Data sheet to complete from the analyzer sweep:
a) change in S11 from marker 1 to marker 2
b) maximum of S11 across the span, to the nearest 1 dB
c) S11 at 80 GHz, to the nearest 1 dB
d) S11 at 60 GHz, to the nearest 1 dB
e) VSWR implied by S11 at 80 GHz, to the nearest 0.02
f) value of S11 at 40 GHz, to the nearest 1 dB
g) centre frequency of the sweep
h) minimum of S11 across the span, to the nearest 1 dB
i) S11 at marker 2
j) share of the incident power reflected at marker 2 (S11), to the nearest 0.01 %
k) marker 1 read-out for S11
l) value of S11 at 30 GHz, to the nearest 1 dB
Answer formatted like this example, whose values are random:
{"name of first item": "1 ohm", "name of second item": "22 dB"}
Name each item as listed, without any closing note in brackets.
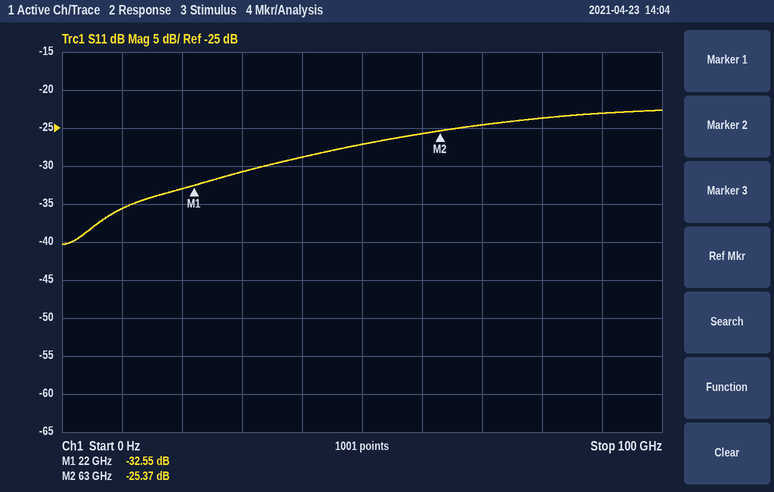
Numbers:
{"change in S11 from marker 1 to marker 2": "7.18 dB", "maximum of S11 across the span, to the nearest 1 dB": "-23 dB", "S11 at 80 GHz, to the nearest 1 dB": "-24 dB", "S11 at 60 GHz, to the nearest 1 dB": "-26 dB", "VSWR implied by S11 at 80 GHz, to the nearest 0.02": "1.14", "value of S11 at 40 GHz, to the nearest 1 dB": "-29 dB", "centre frequency of the sweep": "50 GHz", "minimum of S11 across the span, to the nearest 1 dB": "-40 dB", "S11 at marker 2": "-25.37 dB", "share of the incident power reflected at marker 2 (S11), to the nearest 0.01 %": "0.29 %", "marker 1 read-out for S11": "-32.55 dB", "value of S11 at 30 GHz, to the nearest 1 dB": "-31 dB"}
